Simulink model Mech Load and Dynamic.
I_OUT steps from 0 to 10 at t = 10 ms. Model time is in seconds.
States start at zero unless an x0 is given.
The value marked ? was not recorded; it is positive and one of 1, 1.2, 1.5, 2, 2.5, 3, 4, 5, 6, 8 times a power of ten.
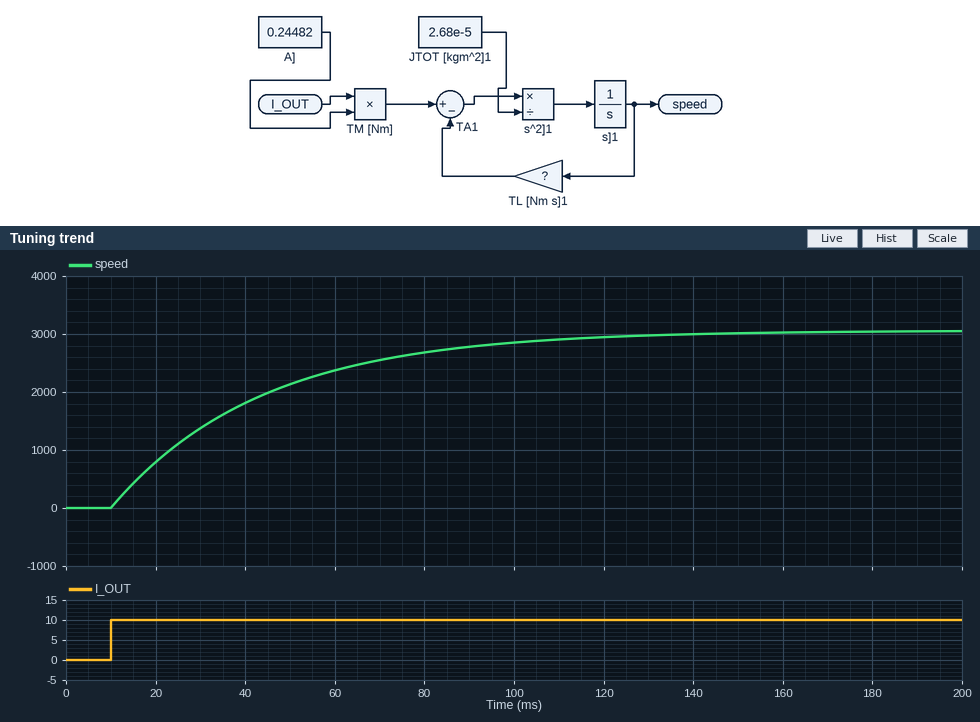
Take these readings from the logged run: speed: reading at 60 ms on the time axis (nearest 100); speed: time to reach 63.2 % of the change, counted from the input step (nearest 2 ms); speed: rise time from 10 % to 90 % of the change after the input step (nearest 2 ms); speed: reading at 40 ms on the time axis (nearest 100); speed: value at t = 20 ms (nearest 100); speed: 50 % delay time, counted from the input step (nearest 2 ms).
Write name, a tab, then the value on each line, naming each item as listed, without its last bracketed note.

speed: reading at 60 ms on the time axis	2400
speed: time to reach 63.2 % of the change, counted from the input step	34 ms
speed: rise time from 10 % to 90 % of the change after the input step	74 ms
speed: reading at 40 ms on the time axis	1800
speed: value at t = 20 ms	800
speed: 50 % delay time, counted from the input step	24 ms
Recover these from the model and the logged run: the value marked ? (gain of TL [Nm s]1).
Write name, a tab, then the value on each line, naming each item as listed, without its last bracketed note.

the value marked ?	0.0008
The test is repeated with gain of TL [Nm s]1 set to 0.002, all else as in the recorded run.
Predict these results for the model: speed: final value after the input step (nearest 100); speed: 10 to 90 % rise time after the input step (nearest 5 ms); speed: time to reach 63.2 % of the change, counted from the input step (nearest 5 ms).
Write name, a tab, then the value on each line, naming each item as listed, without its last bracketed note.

speed: final value after the input step	1200
speed: 10 to 90 % rise time after the input step	30 ms
speed: time to reach 63.2 % of the change, counted from the input step	15 ms
